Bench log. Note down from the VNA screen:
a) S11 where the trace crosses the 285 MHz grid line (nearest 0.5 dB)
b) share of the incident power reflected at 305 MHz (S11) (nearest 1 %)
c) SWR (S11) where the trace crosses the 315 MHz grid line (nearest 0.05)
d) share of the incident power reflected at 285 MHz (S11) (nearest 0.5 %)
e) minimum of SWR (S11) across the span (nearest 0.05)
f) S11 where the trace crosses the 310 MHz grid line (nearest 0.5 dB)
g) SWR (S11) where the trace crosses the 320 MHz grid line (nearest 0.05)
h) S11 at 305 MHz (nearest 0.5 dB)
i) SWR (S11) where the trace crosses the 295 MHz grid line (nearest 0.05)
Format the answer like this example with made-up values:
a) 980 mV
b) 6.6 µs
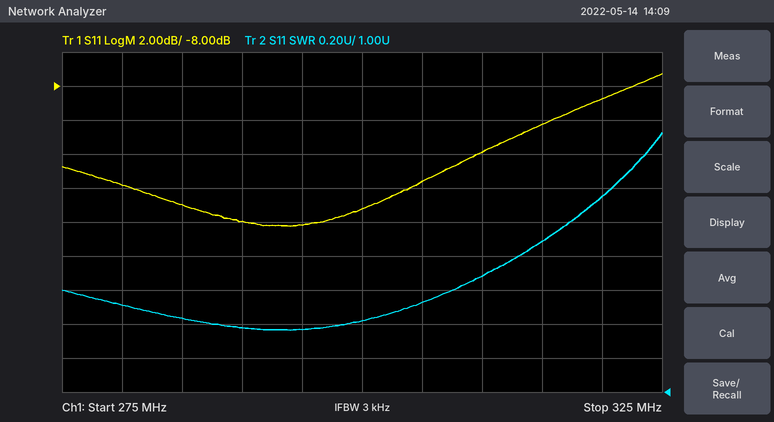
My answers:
a) -15.0 dB
b) 4 %
c) 1.90
d) 3.0 %
e) 1.35
f) -12.0 dB
g) 2.15
h) -13.5 dB
i) 1.35
